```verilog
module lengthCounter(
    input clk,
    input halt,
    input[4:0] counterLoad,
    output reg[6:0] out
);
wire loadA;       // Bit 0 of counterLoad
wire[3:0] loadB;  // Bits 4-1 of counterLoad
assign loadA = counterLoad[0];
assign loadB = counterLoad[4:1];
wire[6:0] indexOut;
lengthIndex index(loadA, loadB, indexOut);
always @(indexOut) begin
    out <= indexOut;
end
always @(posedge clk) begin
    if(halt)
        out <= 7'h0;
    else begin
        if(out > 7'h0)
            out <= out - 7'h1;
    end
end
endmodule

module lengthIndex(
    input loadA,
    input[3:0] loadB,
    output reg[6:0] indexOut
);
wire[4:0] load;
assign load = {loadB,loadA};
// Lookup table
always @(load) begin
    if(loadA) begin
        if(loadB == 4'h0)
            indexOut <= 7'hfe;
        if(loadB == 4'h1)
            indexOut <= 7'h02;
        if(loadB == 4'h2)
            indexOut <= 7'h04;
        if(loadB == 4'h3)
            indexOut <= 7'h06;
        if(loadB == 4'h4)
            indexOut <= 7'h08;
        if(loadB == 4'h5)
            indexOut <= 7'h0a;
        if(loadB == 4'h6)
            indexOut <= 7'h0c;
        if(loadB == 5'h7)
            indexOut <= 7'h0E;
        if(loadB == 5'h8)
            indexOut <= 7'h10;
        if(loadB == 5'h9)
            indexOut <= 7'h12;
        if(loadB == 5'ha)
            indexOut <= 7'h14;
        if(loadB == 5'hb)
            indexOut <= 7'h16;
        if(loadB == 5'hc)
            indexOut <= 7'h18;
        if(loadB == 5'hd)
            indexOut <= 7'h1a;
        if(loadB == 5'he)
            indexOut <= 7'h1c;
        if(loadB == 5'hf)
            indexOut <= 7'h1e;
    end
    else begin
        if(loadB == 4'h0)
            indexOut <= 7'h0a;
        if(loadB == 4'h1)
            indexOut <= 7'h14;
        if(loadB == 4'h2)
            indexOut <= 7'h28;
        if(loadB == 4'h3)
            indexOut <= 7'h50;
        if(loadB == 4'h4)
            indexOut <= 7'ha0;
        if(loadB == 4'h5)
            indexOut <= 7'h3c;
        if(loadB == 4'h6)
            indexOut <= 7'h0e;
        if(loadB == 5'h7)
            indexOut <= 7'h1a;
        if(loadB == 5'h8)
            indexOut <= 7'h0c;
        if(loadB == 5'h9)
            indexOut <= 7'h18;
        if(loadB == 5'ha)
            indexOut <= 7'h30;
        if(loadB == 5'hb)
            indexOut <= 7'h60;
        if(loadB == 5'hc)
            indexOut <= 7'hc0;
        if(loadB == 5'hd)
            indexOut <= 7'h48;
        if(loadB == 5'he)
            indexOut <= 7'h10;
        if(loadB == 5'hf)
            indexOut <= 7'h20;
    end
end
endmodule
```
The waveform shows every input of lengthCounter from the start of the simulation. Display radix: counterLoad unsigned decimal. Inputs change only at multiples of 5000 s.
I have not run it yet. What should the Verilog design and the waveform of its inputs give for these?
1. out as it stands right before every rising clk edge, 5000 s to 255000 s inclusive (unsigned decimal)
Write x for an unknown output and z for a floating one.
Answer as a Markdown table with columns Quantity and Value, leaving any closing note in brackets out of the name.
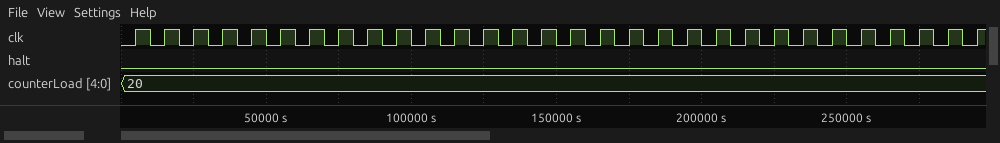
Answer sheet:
| Quantity | Value |
|---|---|
| out as it stands right before every rising clk edge, 5000 s to 255000 s inclusive | 48, 47, 46, 45, 44, 43, 42, 41, 40, 39, 38, 37, 36, 35, 34, 33, 32, 31, 30, 29, 28, 27, 26, 25, 24, 23 |
